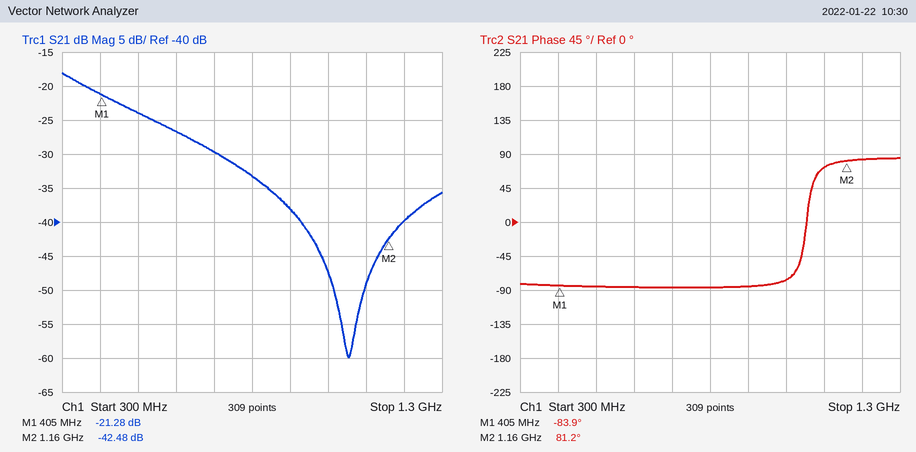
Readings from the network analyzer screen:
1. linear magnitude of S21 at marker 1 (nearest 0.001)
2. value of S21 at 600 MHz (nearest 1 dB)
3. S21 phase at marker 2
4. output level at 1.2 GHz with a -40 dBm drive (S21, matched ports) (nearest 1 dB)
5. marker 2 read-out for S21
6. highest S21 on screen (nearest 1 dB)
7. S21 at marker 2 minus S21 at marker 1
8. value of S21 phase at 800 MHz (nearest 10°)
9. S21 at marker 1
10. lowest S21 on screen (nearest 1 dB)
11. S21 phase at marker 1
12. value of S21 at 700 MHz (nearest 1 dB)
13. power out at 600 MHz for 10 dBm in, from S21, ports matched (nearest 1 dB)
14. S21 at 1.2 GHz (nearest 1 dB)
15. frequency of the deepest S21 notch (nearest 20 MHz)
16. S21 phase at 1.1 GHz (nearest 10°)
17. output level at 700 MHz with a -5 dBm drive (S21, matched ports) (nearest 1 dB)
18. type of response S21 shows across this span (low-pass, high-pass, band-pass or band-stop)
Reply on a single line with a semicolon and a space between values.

0.086; -27 dB; 81.2°; -80 dBm; -42.48 dB; -18 dB; -21.20 dB; -90°; -21.28 dB; -60 dB; -83.9°; -30 dB; -17 dBm; -40 dB; 1.06 GHz; 70°; -35 dBm; low-pass
